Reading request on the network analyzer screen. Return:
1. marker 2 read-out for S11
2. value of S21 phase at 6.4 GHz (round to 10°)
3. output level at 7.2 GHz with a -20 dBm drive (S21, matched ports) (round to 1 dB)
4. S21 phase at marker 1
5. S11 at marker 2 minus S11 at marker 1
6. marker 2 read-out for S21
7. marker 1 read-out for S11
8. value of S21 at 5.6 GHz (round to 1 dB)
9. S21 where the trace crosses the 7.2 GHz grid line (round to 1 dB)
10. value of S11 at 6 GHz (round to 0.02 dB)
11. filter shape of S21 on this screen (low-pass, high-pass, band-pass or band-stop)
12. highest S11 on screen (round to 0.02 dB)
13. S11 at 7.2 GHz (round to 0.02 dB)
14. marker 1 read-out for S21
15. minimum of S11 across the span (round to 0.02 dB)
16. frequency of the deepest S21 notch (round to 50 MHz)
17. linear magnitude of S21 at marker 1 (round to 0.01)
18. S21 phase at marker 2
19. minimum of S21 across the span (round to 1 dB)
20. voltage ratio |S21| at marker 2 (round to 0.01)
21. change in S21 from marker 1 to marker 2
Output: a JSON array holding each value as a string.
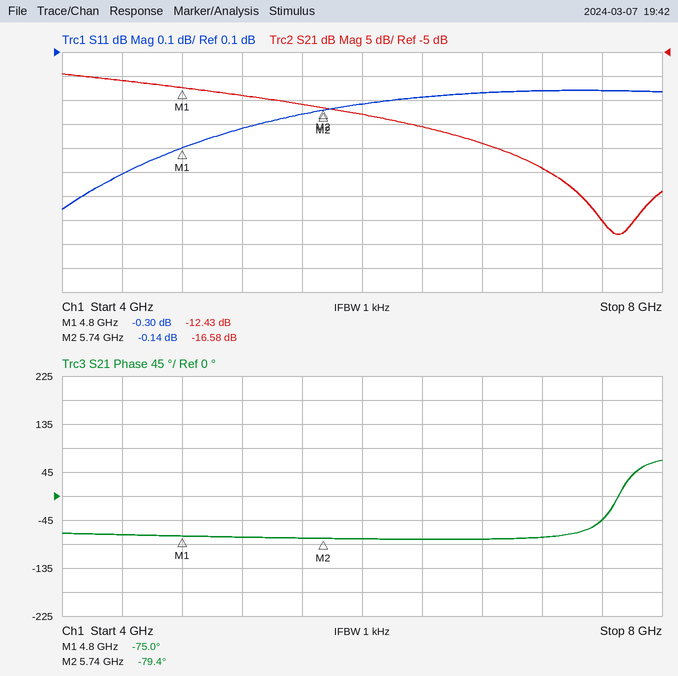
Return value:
["-0.14 dB", "-80°", "-49 dBm", "-75.0°", "0.16 dB", "-16.58 dB", "-0.30 dB", "-16 dB", "-29 dB", "-0.12 dB", "low-pass", "-0.06 dB", "-0.06 dB", "-12.43 dB", "-0.56 dB", "7.70 GHz", "0.24", "-79.4°", "-43 dB", "0.15", "-4.15 dB"]
